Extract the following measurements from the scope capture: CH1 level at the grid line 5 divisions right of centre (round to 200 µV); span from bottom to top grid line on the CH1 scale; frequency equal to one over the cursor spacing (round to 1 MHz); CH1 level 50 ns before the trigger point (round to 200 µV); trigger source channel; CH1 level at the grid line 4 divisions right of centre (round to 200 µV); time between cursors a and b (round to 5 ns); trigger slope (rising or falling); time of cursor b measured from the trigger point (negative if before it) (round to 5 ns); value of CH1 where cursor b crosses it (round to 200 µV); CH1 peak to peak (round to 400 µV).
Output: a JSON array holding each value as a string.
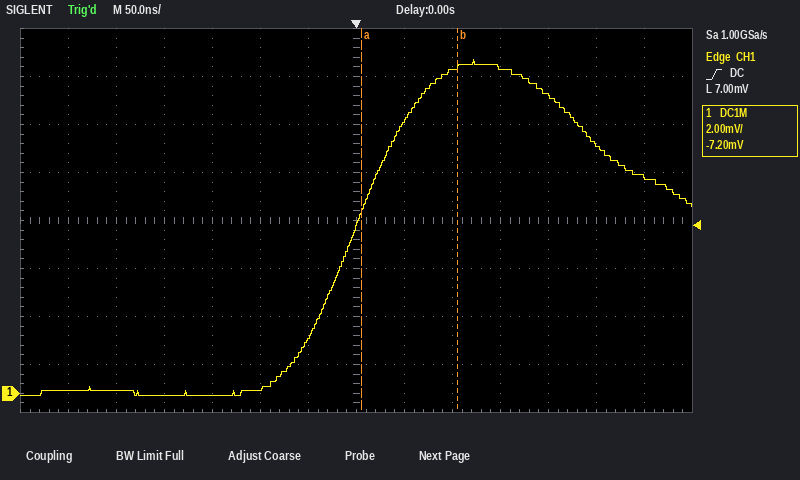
["10.4 mV", "16 mV", "10 MHz", "2.2 mV", "CH1", "12.4 mV", "100 ns", "rising", "+105 ns", "13.6 mV", "14.0 mV"]
